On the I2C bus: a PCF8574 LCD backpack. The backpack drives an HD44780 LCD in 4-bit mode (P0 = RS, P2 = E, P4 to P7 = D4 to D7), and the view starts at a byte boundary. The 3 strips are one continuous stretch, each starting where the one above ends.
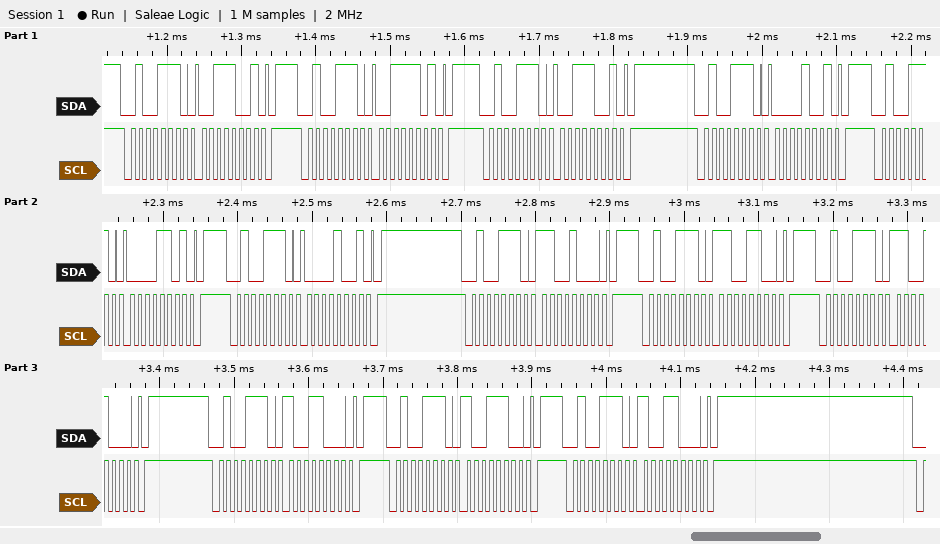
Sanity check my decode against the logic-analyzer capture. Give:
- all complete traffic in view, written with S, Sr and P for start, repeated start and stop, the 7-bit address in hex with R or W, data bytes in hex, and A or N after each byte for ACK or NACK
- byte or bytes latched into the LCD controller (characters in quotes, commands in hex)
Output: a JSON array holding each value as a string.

["S 27W A 39 A P S 27W A 3D A P S 27W A 39 A P S 27W A 09 A P S 27W A 0D A P S 27W A 09 A P S 27W A C8 A P S 27W A CC A P S 27W A C8 A P S 27W A 98 A P S 27W A 9C A P S 27W A 98 A P", "'0' 0xC9"]
